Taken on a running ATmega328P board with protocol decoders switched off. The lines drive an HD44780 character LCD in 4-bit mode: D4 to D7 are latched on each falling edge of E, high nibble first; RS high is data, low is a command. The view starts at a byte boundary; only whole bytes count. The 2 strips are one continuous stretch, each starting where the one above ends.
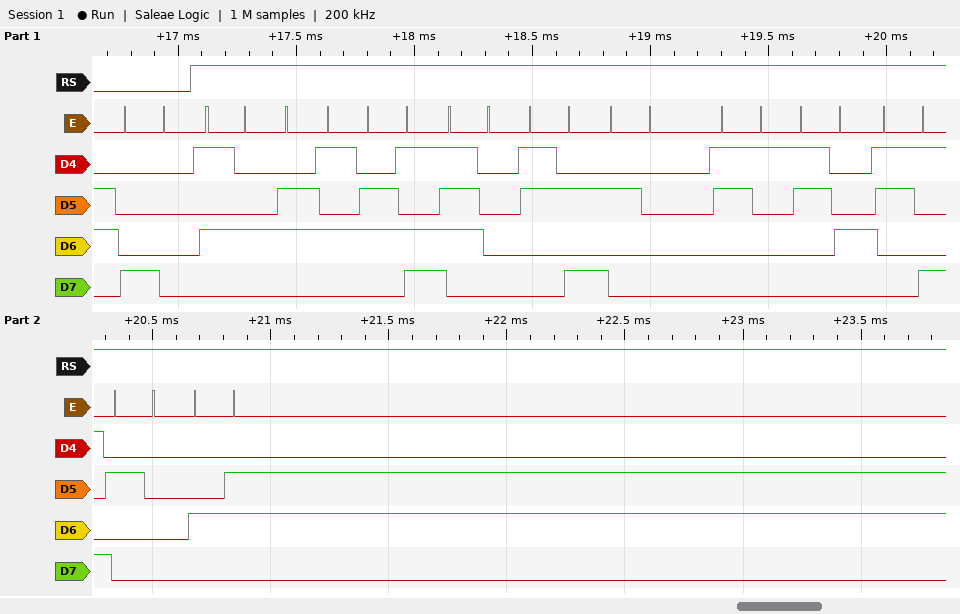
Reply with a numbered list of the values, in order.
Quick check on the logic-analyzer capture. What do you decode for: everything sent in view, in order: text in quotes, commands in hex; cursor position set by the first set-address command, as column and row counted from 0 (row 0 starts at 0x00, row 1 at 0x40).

1. 0x80 "Temp: 149 F"
2. column 0, row 0
